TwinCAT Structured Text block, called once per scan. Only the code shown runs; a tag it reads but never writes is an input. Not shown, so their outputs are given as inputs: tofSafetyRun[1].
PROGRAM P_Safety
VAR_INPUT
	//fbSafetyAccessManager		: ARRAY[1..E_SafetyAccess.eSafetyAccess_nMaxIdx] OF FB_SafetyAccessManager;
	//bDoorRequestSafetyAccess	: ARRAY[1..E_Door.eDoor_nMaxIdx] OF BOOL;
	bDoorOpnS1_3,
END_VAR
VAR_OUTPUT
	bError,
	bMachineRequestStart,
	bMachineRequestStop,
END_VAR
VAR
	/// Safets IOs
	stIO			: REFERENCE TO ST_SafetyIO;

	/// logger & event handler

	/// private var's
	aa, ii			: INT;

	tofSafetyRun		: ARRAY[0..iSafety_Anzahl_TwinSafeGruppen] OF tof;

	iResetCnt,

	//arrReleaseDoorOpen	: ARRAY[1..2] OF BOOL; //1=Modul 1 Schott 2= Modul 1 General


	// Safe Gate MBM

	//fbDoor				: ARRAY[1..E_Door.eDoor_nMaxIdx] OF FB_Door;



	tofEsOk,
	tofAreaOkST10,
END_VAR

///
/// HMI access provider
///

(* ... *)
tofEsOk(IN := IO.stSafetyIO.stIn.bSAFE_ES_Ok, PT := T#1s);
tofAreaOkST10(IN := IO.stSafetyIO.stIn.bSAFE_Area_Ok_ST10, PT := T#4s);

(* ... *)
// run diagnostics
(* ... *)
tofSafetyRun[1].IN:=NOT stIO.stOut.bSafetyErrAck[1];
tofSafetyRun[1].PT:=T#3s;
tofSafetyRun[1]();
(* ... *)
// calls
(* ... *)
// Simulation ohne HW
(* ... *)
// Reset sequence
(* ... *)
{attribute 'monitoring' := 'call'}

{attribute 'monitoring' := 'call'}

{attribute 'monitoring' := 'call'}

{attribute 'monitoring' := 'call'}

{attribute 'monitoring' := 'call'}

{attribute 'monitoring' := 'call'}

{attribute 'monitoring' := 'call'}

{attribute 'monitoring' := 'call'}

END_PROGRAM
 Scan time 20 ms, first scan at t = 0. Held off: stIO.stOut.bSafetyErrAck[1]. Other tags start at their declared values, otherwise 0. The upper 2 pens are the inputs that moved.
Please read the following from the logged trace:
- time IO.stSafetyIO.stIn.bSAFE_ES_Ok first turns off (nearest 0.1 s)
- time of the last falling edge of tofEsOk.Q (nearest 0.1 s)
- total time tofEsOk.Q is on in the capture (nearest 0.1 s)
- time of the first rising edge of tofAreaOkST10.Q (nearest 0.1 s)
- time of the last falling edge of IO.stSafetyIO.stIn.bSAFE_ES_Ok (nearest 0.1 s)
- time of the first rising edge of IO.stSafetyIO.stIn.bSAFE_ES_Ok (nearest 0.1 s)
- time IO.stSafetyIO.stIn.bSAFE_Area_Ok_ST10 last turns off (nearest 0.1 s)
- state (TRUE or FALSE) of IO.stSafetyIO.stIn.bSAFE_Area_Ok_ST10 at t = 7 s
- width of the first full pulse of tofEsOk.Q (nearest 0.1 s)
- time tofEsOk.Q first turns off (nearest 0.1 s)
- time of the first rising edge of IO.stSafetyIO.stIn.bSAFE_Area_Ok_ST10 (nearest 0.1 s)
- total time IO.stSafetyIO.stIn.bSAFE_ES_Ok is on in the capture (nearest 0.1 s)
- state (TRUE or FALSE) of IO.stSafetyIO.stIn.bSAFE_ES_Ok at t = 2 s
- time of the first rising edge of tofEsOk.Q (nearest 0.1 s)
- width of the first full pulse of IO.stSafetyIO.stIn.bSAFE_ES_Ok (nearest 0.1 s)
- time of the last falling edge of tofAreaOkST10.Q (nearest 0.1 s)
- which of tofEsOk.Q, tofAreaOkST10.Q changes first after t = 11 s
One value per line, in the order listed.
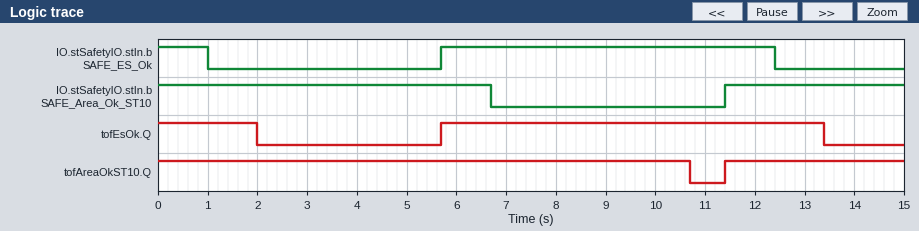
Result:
1.0 s
13.4 s
9.7 s
11.4 s
12.4 s
5.7 s
6.7 s
FALSE
7.7 s
2.0 s
11.4 s
7.7 s
FALSE
5.7 s
6.7 s
10.7 s
tofAreaOkST10.Q
